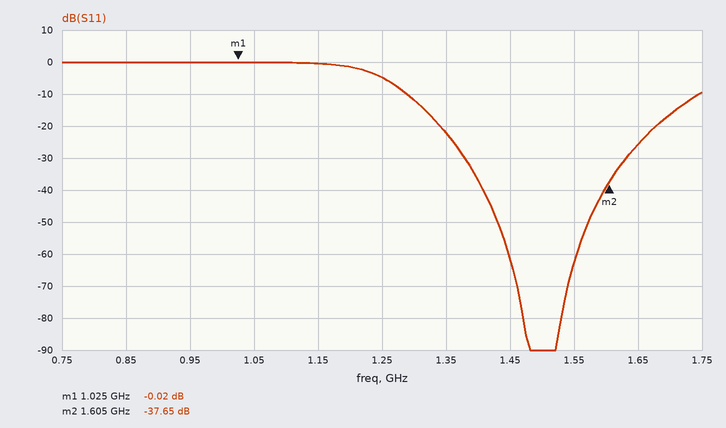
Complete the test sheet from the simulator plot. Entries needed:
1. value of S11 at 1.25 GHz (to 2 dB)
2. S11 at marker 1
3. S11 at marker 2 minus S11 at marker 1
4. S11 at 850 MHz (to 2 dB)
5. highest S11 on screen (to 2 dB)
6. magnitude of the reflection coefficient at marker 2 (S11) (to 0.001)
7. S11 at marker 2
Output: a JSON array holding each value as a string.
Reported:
["-4 dB", "-0.02 dB", "-37.63 dB", "0 dB", "0 dB", "0.013", "-37.65 dB"]
